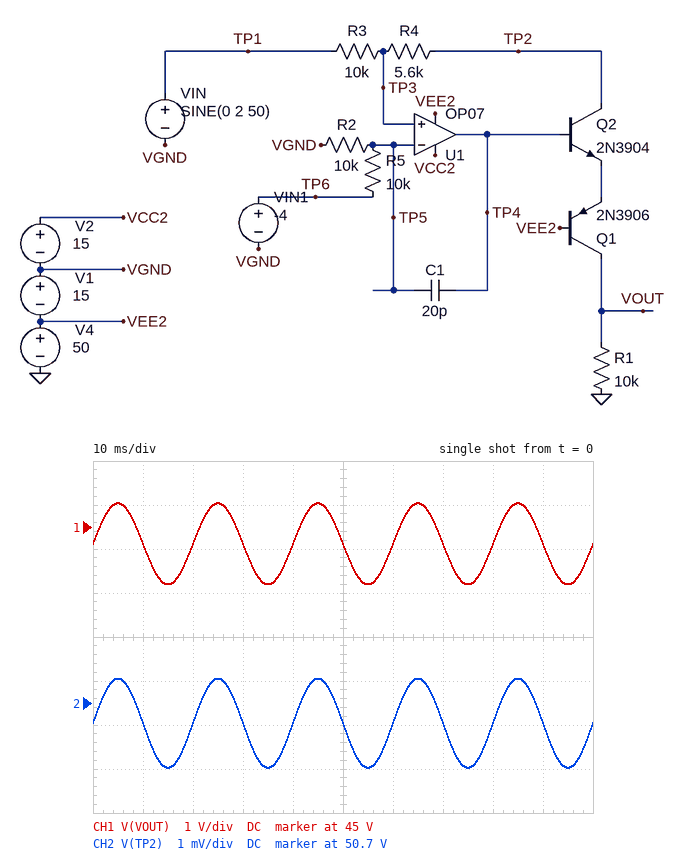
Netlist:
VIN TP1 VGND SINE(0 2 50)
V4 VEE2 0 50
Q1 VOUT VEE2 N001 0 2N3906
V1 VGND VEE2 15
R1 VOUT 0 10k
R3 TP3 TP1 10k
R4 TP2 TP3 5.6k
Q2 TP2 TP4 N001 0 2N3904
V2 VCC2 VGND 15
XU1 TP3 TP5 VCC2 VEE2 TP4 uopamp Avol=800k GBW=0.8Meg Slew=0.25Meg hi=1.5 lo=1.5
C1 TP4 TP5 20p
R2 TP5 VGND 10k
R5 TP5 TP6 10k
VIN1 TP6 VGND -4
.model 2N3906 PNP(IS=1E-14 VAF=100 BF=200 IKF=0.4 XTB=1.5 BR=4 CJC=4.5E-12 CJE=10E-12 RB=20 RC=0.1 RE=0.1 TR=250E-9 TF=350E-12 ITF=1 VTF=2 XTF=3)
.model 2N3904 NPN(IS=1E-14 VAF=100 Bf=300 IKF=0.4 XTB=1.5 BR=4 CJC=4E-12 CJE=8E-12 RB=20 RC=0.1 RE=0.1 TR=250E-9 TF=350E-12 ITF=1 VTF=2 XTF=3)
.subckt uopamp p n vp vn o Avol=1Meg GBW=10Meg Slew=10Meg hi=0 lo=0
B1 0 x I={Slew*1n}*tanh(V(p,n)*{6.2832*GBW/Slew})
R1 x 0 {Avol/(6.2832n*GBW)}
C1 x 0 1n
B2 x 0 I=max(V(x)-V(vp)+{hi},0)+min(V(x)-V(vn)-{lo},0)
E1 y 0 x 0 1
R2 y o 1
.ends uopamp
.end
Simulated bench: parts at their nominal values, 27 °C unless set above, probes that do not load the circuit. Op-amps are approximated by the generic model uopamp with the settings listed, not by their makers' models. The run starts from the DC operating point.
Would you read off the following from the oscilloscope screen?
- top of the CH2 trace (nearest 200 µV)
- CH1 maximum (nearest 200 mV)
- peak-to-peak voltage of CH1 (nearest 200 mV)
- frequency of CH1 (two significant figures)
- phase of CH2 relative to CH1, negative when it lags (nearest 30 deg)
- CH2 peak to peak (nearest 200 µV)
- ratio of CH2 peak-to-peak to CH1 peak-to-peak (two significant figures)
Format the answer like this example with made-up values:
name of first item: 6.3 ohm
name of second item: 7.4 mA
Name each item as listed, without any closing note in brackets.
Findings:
top of the CH2 trace: 50.7026 V
CH1 maximum: 45.6 V
peak-to-peak voltage of CH1: 1.8 V
frequency of CH1: 50 Hz
phase of CH2 relative to CH1, negative when it lags: 0 deg
CH2 peak to peak: 2.0 mV
ratio of CH2 peak-to-peak to CH1 peak-to-peak: 0.0011
